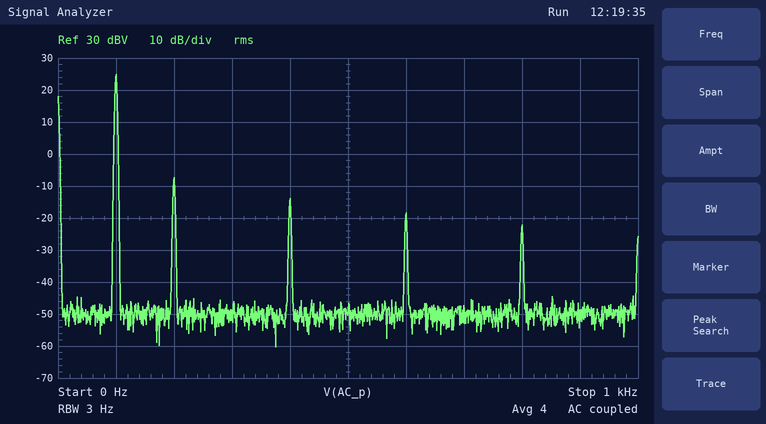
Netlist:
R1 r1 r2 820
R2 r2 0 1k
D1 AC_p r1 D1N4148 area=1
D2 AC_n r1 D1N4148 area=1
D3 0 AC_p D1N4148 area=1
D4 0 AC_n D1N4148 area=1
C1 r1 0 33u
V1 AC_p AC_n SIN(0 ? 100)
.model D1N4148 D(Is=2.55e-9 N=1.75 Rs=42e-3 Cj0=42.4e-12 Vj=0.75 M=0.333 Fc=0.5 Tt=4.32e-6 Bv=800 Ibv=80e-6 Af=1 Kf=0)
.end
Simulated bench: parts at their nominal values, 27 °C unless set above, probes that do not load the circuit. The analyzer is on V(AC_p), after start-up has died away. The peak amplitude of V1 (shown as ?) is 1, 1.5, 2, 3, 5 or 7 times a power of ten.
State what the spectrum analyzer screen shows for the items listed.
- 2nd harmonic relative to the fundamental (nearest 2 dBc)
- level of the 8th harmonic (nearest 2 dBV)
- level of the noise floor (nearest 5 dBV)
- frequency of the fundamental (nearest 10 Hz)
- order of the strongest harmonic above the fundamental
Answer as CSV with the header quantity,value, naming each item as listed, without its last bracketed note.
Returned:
quantity,value
2nd harmonic relative to the fundamental,-32 dBc
level of the 8th harmonic,-22 dBV
level of the noise floor,-50 dBV
frequency of the fundamental,100 Hz
order of the strongest harmonic above the fundamental,2
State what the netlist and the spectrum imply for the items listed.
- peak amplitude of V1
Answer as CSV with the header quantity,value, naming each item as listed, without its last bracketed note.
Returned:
quantity,value
peak amplitude of V1,50 V
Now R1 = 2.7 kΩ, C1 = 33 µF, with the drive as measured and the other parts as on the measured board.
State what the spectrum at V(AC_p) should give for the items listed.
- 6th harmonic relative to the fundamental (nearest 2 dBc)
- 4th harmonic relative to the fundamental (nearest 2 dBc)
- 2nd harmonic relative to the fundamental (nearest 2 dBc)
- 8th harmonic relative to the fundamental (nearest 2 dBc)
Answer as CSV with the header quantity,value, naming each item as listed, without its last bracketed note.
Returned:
quantity,value
6th harmonic relative to the fundamental,-48 dBc
4th harmonic relative to the fundamental,-44 dBc
2nd harmonic relative to the fundamental,-38 dBc
8th harmonic relative to the fundamental,-52 dBc
